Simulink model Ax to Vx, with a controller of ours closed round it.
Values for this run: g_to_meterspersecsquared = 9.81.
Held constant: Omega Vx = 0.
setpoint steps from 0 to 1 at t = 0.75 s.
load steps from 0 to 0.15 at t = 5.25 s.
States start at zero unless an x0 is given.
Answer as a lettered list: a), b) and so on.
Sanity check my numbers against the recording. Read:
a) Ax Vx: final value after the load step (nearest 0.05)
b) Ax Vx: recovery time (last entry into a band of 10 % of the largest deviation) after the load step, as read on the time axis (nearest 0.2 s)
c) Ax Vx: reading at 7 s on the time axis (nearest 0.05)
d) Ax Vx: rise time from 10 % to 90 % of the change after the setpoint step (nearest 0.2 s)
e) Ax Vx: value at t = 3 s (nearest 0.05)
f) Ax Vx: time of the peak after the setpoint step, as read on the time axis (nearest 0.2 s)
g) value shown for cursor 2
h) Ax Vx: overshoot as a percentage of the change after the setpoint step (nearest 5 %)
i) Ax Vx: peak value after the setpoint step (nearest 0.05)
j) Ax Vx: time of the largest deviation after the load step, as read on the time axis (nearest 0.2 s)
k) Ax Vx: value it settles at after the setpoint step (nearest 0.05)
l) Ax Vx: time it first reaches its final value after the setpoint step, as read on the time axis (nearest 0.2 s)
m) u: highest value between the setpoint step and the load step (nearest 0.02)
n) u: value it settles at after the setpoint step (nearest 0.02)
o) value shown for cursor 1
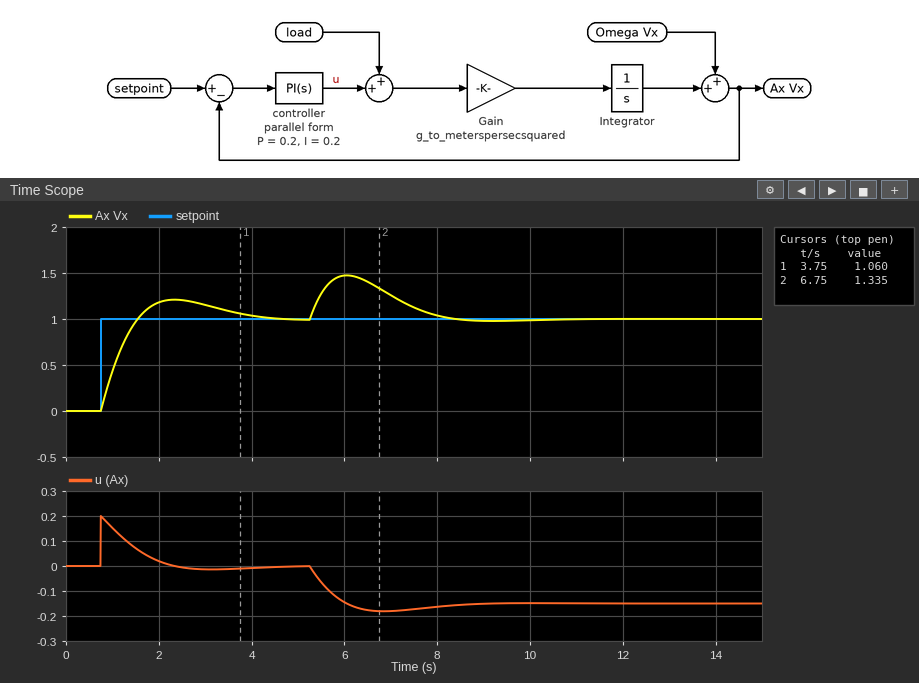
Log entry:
a) 1.00
b) 8.0 s
c) 1.25
d) 0.6 s
e) 1.15
f) 2.4 s
g) 1.335
h) 20 %
i) 1.20
j) 6.0 s
k) 1.00
l) 1.6 s
m) 0.20
n) 0.00
o) 1.060
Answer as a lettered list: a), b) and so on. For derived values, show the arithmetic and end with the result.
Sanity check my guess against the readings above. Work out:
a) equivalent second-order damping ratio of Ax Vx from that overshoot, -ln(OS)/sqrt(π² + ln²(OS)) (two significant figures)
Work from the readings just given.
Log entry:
a) ln(0.2) = -1.609; 1.609 / sqrt(9.870 + 2.590) = 0.46
